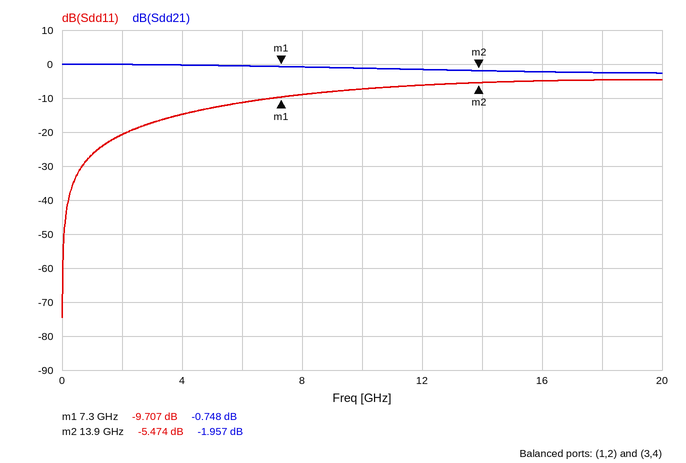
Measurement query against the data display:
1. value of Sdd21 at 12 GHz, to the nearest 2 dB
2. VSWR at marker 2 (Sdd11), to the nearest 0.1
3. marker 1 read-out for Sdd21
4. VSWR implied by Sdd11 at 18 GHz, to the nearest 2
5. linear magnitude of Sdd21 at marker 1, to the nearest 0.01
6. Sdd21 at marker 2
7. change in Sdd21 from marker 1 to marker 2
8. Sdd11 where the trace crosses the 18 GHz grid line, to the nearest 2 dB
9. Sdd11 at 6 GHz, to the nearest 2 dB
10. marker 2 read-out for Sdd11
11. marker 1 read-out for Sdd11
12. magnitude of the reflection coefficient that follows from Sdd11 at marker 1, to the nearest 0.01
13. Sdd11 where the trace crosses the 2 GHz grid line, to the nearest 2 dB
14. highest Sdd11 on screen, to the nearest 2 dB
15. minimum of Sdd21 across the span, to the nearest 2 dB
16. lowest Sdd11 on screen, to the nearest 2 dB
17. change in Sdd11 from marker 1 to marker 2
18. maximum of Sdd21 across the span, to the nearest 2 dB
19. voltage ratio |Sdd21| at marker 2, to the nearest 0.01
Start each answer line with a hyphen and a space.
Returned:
- -2 dB
- 3.3
- -0.748 dB
- 4
- 0.92
- -1.957 dB
- -1.209 dB
- -4 dB
- -12 dB
- -5.474 dB
- -9.707 dB
- 0.33
- -20 dB
- -4 dB
- -2 dB
- -74 dB
- 4.233 dB
- 0 dB
- 0.80
